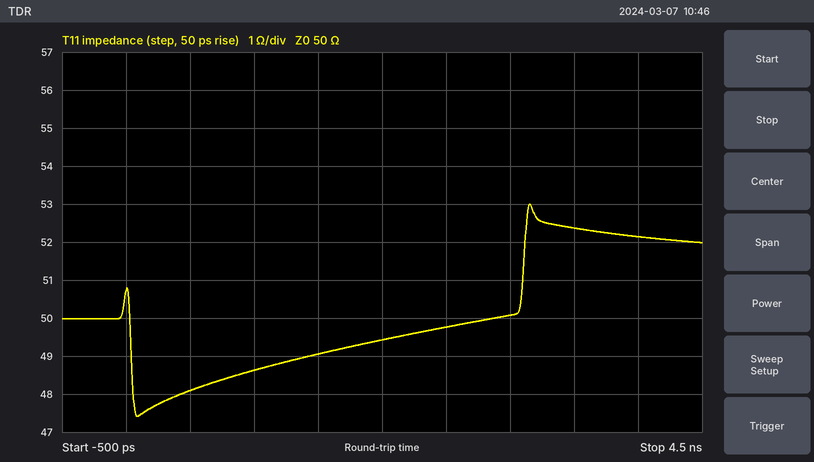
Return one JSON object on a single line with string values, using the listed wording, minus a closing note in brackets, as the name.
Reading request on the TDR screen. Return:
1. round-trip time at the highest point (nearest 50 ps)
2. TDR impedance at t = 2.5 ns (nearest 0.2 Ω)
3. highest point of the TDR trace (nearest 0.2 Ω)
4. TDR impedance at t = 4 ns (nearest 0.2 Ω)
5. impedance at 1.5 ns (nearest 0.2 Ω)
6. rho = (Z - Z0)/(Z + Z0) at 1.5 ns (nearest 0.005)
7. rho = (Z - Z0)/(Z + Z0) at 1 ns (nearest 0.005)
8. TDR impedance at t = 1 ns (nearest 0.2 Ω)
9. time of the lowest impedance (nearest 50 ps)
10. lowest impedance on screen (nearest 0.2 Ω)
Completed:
{"round-trip time at the highest point": "3.15 ns", "TDR impedance at t = 2.5 ns": "49.8 Ω", "highest point of the TDR trace": "53.0 Ω", "TDR impedance at t = 4 ns": "52.2 Ω", "impedance at 1.5 ns": "49.0 Ω", "rho = (Z - Z0)/(Z + Z0) at 1.5 ns": "-0.010", "rho = (Z - Z0)/(Z + Z0) at 1 ns": "-0.015", "TDR impedance at t = 1 ns": "48.6 Ω", "time of the lowest impedance": "100 ps", "lowest impedance on screen": "47.4 Ω"}
